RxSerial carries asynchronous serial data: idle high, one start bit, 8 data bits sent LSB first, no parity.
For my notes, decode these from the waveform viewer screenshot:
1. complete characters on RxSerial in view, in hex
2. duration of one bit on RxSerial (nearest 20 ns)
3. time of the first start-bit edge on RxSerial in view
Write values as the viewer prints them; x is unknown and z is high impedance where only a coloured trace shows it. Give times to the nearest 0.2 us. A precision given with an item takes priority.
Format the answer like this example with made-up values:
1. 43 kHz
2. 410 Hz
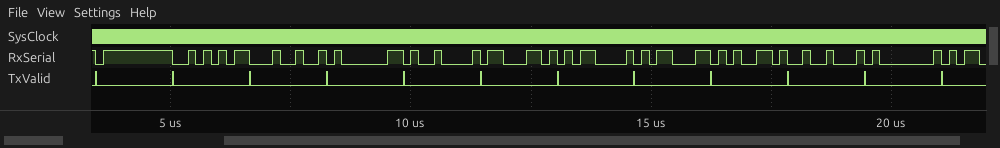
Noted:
1. FF, AA, 24, 81, 09, 63, 0D, 8D, 65, 12, 01
2. 160 ns
3. 3.4 us
